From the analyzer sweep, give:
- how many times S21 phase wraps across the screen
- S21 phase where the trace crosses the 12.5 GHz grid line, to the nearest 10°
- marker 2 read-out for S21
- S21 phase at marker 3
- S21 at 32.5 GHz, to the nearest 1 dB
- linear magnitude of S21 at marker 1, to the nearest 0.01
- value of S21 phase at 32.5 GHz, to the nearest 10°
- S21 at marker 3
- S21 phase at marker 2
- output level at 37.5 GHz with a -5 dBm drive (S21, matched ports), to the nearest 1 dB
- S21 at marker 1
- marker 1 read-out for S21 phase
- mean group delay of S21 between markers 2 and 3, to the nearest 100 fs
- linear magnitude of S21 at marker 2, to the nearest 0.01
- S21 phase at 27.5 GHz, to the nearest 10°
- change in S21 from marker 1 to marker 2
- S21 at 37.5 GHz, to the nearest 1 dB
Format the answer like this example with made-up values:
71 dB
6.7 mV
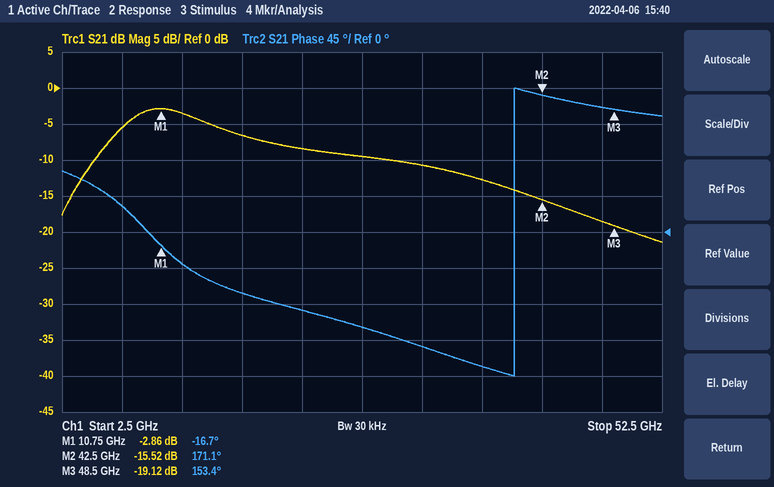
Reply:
1
-40°
-15.52 dB
153.4°
-11 dB
0.72
-140°
-19.12 dB
171.1°
-18 dBm
-2.86 dB
-16.7°
8.2 ps
0.17
-120°
-12.66 dB
-13 dB
